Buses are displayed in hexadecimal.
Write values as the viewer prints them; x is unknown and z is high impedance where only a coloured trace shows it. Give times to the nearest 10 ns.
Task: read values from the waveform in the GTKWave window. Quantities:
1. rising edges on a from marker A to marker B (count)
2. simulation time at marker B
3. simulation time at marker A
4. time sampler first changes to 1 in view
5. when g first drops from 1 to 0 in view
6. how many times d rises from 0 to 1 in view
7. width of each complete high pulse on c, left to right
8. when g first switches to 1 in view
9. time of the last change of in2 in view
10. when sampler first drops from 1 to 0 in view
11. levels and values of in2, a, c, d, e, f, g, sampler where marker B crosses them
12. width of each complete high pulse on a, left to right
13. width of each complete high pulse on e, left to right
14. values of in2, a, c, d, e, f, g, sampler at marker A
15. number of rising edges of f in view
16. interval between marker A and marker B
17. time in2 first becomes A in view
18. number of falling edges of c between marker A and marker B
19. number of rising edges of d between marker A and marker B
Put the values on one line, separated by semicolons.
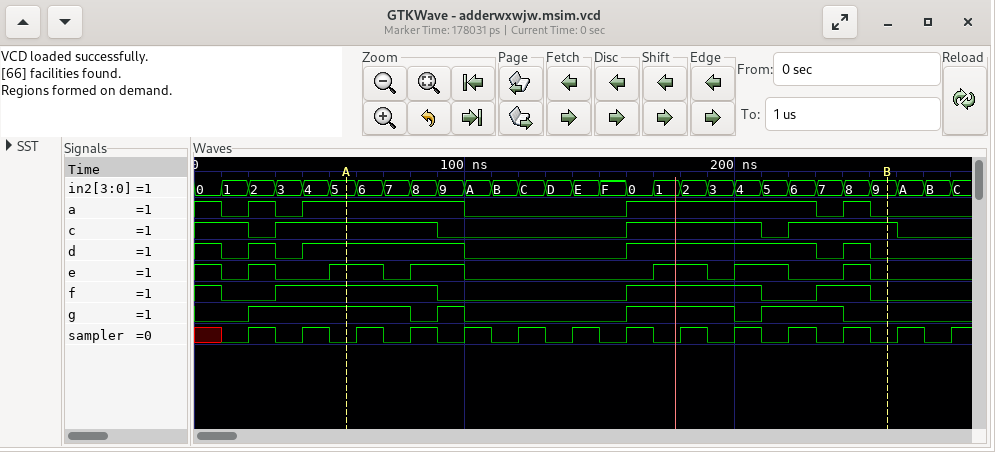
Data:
2; 260 ns; 60 ns; 20 ns; 80 ns; 4; 60 ns, 50 ns, 40 ns; 20 ns; 280 ns; 30 ns; in2=9, a=0, c=1, d=0, e=0, f=0, g=0, sampler=0; 10 ns, 60 ns, 70 ns, 10 ns; 10 ns, 20 ns, 20 ns, 20 ns, 20 ns, 10 ns; in2=5, a=1, c=1, d=1, e=1, f=1, g=1, sampler=0; 3; 200 ns; 100 ns; 2; 2
